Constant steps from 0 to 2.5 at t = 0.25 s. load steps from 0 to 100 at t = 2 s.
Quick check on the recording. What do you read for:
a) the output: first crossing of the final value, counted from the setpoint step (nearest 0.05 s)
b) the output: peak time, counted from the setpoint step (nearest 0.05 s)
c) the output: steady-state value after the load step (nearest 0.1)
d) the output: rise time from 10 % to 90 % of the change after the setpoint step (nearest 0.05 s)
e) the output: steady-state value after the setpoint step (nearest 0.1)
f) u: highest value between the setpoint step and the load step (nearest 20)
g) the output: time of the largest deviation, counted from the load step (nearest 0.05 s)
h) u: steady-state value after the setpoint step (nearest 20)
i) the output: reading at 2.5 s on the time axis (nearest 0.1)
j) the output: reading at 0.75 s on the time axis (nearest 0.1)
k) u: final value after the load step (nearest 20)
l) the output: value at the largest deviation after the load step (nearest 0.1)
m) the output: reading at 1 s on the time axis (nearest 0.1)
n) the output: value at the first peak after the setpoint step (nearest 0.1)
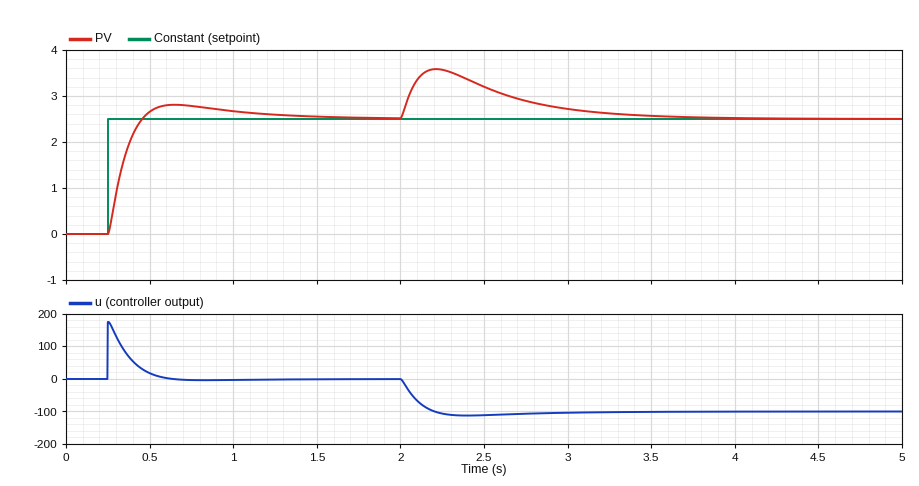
0.20 s
0.40 s
2.5
0.15 s
2.5
180
0.20 s
0
3.2
2.8
-100
3.6
2.7
2.8
